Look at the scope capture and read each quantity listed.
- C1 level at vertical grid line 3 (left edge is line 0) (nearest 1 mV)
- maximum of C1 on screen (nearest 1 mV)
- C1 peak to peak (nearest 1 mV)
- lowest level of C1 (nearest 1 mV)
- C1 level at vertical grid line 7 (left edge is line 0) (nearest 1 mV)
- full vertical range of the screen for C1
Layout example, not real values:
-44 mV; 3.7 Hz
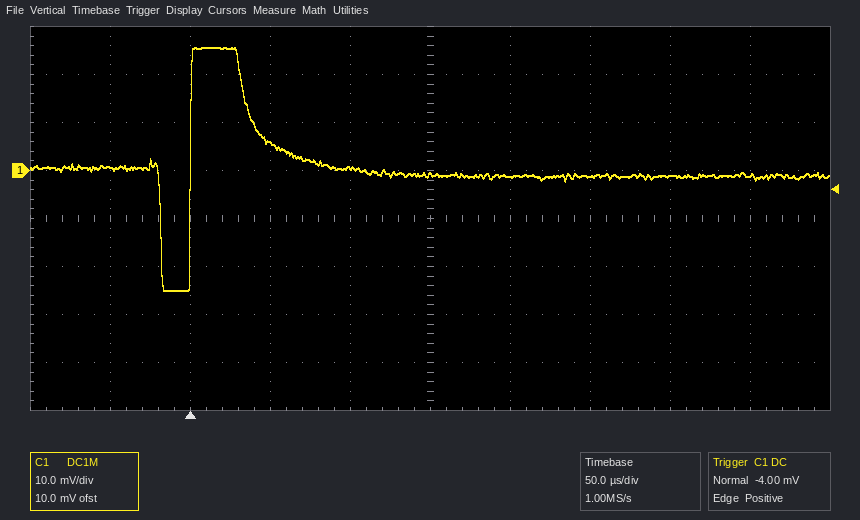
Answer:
6 mV; 26 mV; 51 mV; -25 mV; -1 mV; 80 mV
